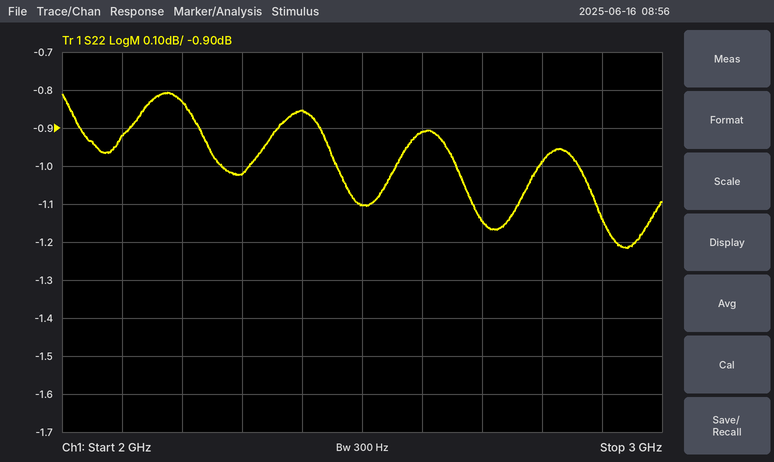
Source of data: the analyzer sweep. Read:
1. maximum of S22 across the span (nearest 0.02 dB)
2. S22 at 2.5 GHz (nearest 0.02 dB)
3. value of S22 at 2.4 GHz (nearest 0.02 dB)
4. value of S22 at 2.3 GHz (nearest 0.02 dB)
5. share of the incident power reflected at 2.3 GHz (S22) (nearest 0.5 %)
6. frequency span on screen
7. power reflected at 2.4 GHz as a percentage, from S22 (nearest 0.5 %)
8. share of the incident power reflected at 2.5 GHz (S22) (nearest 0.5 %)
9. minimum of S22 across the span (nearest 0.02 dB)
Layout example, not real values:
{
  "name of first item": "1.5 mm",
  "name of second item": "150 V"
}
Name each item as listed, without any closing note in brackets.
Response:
{
  "maximum of S22 across the span": "-0.80 dB",
  "S22 at 2.5 GHz": "-1.10 dB",
  "value of S22 at 2.4 GHz": "-0.86 dB",
  "value of S22 at 2.3 GHz": "-1.02 dB",
  "share of the incident power reflected at 2.3 GHz (S22)": "79.0 %",
  "frequency span on screen": "1 GHz",
  "power reflected at 2.4 GHz as a percentage, from S22": "82.0 %",
  "share of the incident power reflected at 2.5 GHz (S22)": "77.5 %",
  "minimum of S22 across the span": "-1.22 dB"
}
